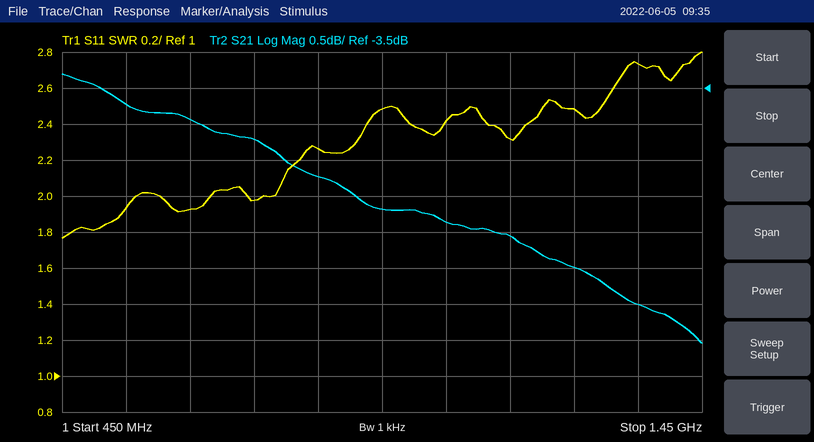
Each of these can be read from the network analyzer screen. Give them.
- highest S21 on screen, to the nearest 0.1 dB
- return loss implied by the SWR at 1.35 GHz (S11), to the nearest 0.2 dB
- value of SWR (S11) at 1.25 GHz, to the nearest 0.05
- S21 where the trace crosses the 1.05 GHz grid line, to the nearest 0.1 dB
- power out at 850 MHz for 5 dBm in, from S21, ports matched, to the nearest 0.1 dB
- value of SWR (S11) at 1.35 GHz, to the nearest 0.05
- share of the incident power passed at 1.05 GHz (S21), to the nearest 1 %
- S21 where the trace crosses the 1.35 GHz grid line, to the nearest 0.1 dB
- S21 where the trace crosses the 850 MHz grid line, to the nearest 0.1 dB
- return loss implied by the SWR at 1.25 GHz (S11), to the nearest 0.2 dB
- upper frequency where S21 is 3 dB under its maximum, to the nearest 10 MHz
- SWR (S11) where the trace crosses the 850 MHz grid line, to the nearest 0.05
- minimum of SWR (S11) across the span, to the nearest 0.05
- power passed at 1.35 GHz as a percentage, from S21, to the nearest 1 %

-3.3 dB
6.6 dB
2.50
-5.4 dB
0.3 dBm
2.75
29 %
-6.5 dB
-4.7 dB
7.4 dB
1.31 GHz
2.25
1.75
22 %
